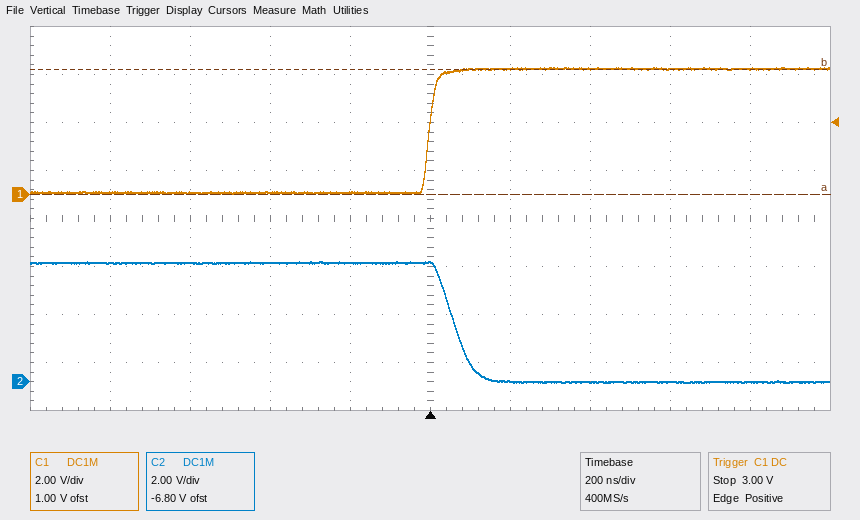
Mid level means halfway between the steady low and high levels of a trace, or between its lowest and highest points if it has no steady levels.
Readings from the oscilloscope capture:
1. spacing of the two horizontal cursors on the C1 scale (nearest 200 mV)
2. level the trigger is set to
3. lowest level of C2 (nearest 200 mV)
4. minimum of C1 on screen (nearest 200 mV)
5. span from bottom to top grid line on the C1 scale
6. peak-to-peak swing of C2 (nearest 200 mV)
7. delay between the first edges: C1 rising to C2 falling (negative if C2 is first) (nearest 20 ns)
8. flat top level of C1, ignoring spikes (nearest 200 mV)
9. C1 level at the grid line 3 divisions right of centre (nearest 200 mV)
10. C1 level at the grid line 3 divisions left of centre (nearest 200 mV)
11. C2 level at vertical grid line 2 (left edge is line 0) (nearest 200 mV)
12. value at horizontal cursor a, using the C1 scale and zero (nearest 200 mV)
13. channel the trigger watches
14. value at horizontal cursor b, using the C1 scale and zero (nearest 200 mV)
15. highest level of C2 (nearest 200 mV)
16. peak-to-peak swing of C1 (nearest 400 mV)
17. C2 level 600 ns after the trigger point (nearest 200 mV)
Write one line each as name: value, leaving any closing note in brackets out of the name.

spacing of the two horizontal cursors on the C1 scale: 5.2 V
level the trigger is set to: 3.00 V
lowest level of C2: 0.0 V
minimum of C1 on screen: 0.0 V
span from bottom to top grid line on the C1 scale: 16 V
peak-to-peak swing of C2: 5.0 V
delay between the first edges: C1 rising to C2 falling (negative if C2 is first): +60 ns
flat top level of C1, ignoring spikes: 5.2 V
C1 level at the grid line 3 divisions right of centre: 5.2 V
C1 level at the grid line 3 divisions left of centre: 0.0 V
C2 level at vertical grid line 2 (left edge is line 0): 5.0 V
value at horizontal cursor a, using the C1 scale and zero: 0.0 V
channel the trigger watches: C1
value at horizontal cursor b, using the C1 scale and zero: 5.2 V
highest level of C2: 5.0 V
peak-to-peak swing of C1: 5.2 V
C2 level 600 ns after the trigger point: 0.0 V
